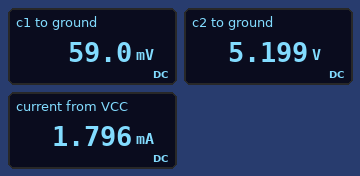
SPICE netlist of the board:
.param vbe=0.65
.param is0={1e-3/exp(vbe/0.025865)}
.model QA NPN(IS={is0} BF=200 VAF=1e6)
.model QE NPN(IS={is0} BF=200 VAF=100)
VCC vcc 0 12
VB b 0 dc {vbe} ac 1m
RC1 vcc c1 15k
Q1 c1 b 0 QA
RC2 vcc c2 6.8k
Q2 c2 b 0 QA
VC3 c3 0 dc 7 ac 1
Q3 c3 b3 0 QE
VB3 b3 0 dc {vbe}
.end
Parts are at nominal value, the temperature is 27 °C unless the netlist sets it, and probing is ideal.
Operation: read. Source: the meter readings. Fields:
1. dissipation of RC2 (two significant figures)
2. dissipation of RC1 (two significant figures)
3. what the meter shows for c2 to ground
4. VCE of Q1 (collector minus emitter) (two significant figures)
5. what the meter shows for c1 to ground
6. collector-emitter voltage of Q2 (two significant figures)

6.8 mW
9.5 mW
5.199 V
59 mV
59.0 mV
5.2 V
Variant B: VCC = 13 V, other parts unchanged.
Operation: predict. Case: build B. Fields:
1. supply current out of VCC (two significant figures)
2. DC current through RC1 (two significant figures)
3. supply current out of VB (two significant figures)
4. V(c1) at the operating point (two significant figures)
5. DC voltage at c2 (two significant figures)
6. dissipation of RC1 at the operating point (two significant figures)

1.9 mA
860 µA
79 µA
69 mV
6.2 V
11 mW
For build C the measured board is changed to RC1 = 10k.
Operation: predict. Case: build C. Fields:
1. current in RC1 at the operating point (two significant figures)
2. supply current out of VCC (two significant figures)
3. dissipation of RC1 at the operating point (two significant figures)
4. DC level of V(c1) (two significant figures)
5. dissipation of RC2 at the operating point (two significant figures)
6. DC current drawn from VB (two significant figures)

1.0 mA
2.0 mA
10 mW
2.0 V
6.8 mW
10 µA
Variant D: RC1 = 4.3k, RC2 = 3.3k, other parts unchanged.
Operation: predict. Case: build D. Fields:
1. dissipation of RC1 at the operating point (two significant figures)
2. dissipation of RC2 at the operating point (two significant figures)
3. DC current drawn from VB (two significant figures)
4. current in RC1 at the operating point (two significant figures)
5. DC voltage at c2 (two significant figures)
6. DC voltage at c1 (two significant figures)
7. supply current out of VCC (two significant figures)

4.3 mW
3.3 mW
10 µA
1.0 mA
8.7 V
7.7 V
2.0 mA
